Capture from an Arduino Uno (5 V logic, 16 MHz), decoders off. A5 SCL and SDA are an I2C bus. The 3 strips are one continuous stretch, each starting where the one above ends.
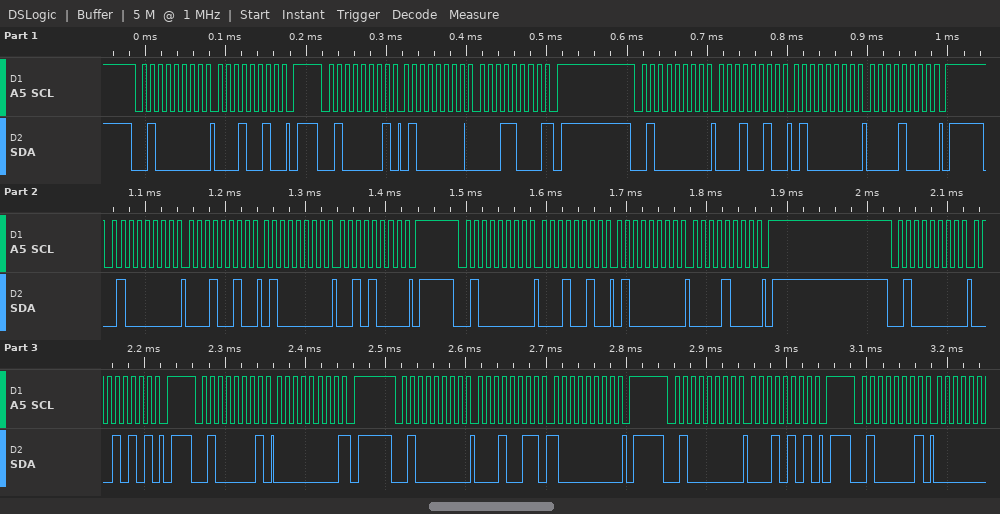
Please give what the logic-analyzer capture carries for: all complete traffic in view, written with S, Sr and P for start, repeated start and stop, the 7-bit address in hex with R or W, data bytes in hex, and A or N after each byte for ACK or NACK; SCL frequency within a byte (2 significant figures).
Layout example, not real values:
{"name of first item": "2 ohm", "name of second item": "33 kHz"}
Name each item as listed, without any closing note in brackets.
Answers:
{"all complete traffic in view, written with S, Sr and P for start, repeated start and stop, the 7-bit address in hex with R or W, data bytes in hex, and A or N after each byte for ACK or NACK": "S 20W A 12 A P S 20R A 40 A 18 N P S 20W A 12 A 40 A 08 A P S 20W A 12 A 40 A 28 A P S 20W A 12 A 40 A 08 A P S 20W A 15 A P S 20R A 00 N P S 20W A 13 A 80 A P S 20W A 15 A P S 20R A", "SCL frequency within a byte": "100 kHz"}
